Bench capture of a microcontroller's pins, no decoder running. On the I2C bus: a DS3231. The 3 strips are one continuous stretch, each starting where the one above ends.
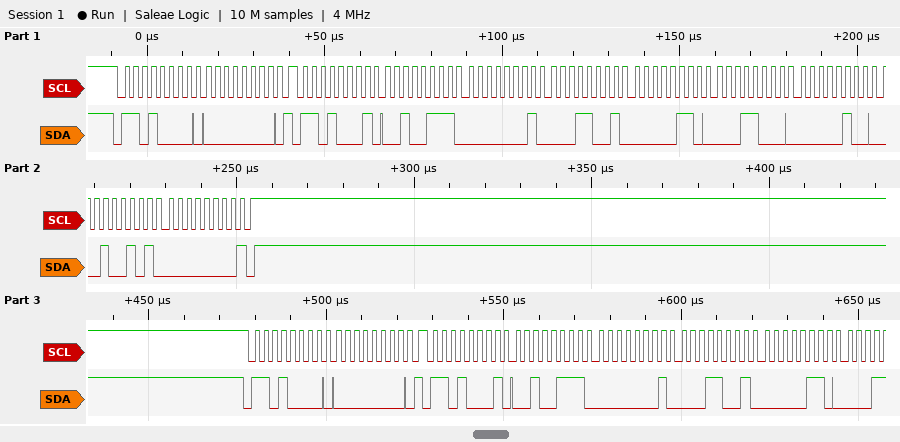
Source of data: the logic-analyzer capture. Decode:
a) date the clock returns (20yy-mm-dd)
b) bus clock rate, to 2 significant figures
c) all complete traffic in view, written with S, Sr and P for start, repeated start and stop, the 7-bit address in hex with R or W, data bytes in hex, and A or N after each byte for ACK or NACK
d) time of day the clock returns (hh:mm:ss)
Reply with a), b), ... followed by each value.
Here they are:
a) 2025-04-18
b) 400 kHz
c) S 68W A 00 A Sr 68R A 27 A 01 A 19 A 06 A 18 A 04 A 25 A 00 N P S 68W A 00 A Sr 68R A 27 A 01 A 19 A 06 A
d) 19:01:27
